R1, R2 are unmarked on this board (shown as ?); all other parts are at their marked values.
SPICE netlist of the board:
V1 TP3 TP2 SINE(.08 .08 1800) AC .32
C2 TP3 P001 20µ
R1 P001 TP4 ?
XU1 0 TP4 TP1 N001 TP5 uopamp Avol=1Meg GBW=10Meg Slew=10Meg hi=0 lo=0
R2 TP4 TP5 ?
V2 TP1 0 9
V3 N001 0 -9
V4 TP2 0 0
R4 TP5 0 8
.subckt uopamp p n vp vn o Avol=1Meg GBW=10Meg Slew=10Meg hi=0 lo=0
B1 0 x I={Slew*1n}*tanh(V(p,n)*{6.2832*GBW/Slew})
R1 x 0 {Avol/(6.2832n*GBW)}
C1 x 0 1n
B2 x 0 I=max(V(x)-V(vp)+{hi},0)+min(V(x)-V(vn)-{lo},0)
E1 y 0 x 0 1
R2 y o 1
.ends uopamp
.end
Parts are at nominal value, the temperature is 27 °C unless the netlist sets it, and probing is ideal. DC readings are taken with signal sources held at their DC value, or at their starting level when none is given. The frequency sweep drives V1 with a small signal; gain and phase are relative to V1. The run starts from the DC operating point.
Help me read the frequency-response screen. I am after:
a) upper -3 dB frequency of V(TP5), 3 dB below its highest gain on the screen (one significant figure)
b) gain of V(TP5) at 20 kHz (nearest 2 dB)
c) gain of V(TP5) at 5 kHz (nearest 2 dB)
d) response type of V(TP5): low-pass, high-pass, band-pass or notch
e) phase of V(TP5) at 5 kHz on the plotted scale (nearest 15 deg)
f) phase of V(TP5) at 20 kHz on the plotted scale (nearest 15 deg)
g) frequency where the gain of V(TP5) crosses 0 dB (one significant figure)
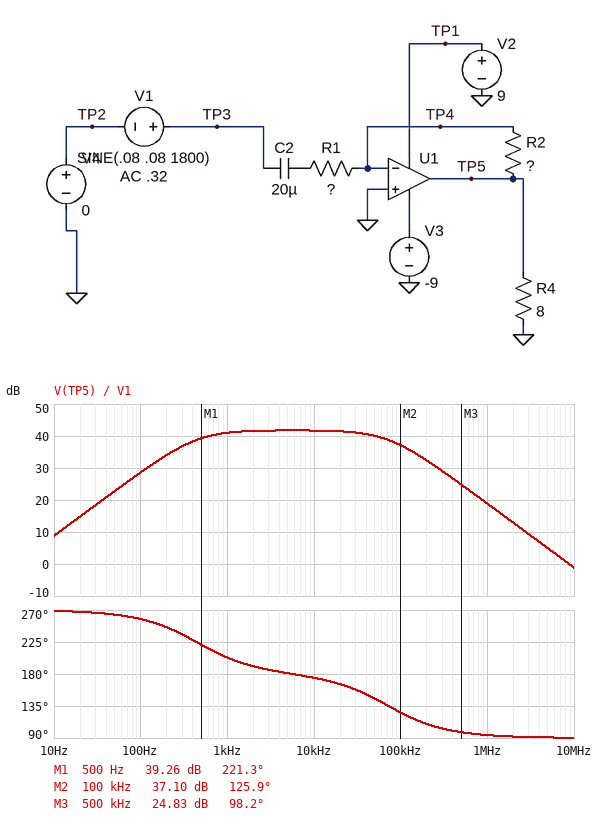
70 kHz
42 dB
42 dB
band-pass
180 deg
165 deg
9 MHz
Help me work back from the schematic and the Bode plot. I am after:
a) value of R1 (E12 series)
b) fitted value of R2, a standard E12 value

18 Ω
2.2 kΩ
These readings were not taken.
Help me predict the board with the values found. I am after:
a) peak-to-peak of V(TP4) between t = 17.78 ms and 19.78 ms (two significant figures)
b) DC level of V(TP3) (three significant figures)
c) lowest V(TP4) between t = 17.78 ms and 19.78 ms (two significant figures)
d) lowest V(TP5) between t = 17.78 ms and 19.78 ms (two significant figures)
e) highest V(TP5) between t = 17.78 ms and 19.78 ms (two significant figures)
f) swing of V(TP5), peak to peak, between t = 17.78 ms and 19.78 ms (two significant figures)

26 mV
80.0 mV
-13 mV
-8.0 V
8.0 V
16 V
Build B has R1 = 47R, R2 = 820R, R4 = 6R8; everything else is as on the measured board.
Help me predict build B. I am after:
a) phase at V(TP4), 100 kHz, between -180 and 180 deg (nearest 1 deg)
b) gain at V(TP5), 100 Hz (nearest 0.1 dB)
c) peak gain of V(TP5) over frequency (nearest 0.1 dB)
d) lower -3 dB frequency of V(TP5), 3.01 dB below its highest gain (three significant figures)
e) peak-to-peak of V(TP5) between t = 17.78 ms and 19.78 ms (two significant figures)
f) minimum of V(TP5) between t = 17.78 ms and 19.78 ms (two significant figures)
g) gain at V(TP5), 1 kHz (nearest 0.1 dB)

78 deg
19.0 dB
24.8 dB
169 Hz
2.8 V
-1.4 V
24.7 dB
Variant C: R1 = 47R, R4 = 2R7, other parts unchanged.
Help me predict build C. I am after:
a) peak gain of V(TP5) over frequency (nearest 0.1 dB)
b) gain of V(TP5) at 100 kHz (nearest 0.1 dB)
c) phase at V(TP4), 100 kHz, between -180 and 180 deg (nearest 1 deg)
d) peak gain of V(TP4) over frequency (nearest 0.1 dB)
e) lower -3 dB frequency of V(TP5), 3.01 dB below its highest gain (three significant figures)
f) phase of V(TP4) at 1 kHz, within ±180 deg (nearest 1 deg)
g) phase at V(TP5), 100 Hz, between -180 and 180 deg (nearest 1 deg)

33.4 dB
31.9 dB
57 deg
-0.2 dB
169 Hz
99 deg
-121 deg
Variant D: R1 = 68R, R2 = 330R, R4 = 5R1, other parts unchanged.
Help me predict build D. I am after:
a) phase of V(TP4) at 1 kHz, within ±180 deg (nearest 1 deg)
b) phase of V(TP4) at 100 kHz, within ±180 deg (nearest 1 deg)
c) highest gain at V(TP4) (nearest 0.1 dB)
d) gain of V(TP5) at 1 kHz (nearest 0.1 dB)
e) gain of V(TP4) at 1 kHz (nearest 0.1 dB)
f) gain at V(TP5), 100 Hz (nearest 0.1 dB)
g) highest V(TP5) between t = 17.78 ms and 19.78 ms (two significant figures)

96 deg
86 deg
-1.6 dB
13.7 dB
-64.8 dB
10.0 dB
390 mV
